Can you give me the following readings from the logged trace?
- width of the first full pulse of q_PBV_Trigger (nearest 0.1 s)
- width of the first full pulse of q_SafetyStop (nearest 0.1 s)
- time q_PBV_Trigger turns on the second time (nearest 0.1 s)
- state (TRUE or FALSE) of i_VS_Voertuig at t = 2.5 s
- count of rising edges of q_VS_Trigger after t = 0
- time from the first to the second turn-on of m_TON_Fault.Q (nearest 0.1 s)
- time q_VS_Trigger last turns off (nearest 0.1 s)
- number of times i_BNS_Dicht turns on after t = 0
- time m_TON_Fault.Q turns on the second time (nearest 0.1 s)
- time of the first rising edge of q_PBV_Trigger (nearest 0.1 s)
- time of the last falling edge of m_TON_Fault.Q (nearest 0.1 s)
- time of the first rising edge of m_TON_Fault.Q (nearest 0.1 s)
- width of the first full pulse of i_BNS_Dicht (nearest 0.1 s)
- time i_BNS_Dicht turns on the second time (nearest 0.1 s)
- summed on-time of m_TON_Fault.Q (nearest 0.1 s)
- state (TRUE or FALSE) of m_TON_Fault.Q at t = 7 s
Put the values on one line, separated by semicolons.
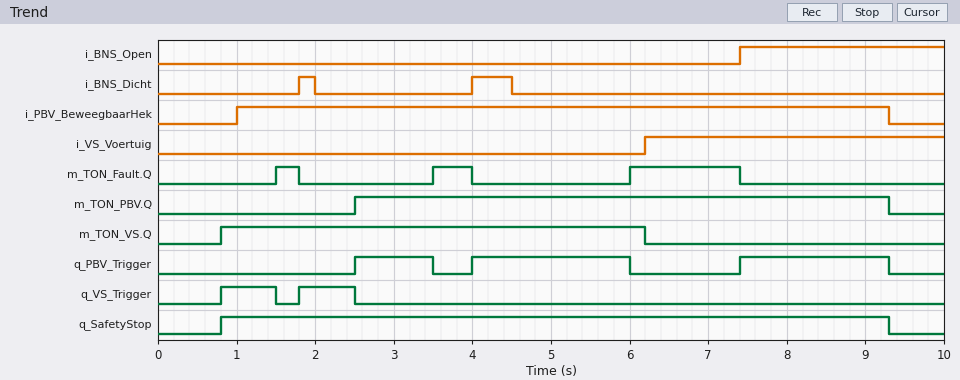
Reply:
1.0 s; 8.5 s; 4.0 s; FALSE; 2; 2.0 s; 2.5 s; 2; 3.5 s; 2.5 s; 7.4 s; 1.5 s; 0.2 s; 4.0 s; 2.2 s; TRUE
